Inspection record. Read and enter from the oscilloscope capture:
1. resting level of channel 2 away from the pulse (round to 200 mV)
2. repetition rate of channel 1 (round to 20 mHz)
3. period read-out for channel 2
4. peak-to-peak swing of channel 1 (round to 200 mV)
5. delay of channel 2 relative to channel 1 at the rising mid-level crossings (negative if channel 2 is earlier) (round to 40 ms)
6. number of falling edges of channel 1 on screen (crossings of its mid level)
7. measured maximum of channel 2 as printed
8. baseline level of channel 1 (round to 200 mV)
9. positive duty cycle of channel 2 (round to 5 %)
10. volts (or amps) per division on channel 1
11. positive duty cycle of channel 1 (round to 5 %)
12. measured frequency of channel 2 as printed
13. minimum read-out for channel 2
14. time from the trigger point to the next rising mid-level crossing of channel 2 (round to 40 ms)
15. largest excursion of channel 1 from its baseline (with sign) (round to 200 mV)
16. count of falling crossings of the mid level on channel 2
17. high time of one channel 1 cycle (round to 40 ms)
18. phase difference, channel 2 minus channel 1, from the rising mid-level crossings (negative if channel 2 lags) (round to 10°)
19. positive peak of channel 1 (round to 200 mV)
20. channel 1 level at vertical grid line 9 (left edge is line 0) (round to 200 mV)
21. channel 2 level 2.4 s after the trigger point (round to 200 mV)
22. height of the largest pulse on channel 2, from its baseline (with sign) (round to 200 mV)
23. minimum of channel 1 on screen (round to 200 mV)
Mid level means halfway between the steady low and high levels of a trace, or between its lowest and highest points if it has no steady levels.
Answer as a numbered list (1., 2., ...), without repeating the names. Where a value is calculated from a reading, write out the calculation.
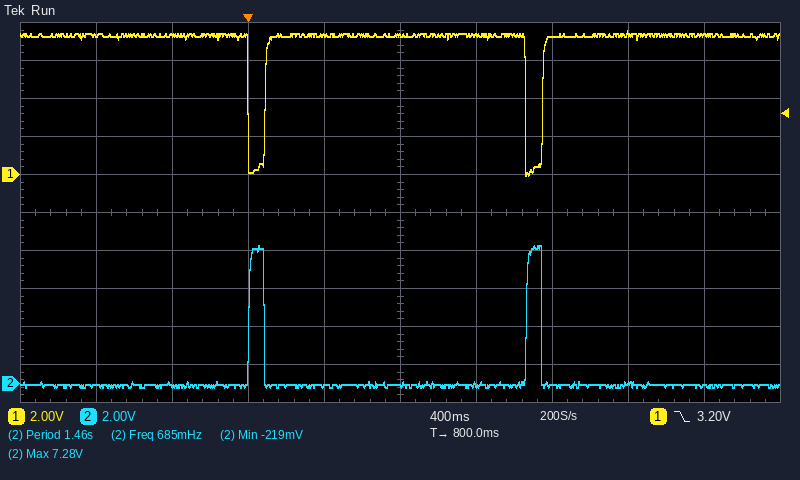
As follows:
1. 0.0 V
2. 680 mHz
3. 1.46 s
4. 7.6 V − (0.0 V) = 7.6 V
5. -80 ms
6. 2
7. 7.28 V
8. 7.4 V
9. 5 %
10. 2 V
11. 95 %
12. 685 mHz
13. -219 mV
14. 1.48 s
15. 0.0 V − (7.4 V) = -7.4 V
16. 2
17. 1.36 s
18. +20°
19. 7.6 V
20. 7.4 V
21. -200 mV
22. +7.4 V
23. 0.0 V
